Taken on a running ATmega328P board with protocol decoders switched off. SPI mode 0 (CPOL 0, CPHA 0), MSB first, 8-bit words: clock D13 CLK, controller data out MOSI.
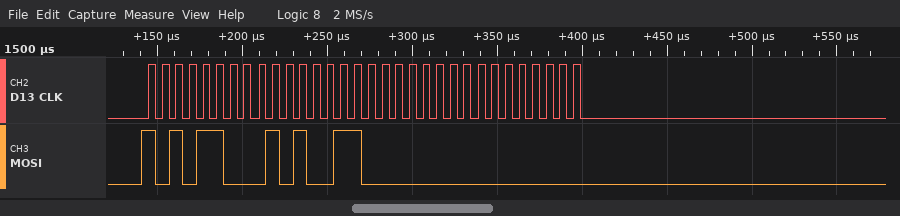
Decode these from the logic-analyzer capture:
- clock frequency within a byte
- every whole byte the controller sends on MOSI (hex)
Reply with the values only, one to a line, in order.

125 kHz
AC 53 00 00
